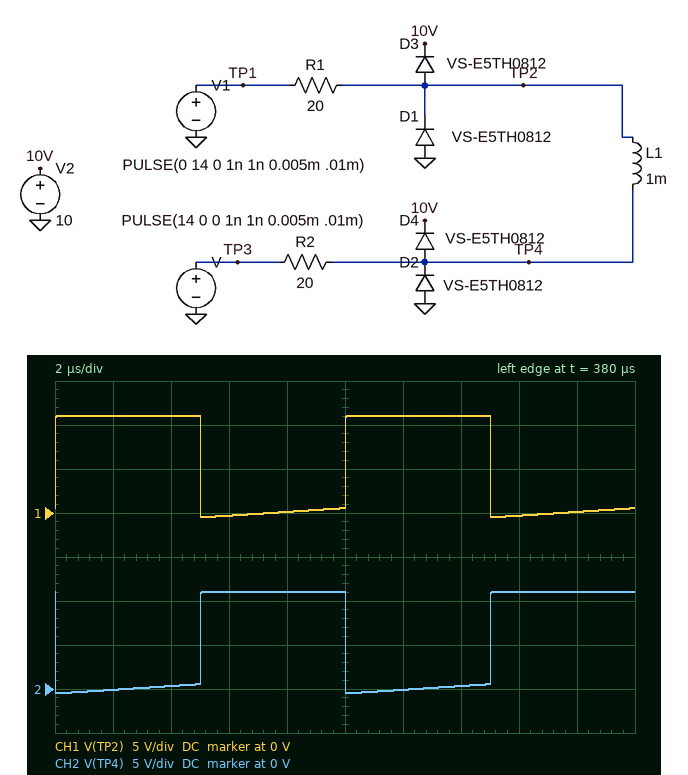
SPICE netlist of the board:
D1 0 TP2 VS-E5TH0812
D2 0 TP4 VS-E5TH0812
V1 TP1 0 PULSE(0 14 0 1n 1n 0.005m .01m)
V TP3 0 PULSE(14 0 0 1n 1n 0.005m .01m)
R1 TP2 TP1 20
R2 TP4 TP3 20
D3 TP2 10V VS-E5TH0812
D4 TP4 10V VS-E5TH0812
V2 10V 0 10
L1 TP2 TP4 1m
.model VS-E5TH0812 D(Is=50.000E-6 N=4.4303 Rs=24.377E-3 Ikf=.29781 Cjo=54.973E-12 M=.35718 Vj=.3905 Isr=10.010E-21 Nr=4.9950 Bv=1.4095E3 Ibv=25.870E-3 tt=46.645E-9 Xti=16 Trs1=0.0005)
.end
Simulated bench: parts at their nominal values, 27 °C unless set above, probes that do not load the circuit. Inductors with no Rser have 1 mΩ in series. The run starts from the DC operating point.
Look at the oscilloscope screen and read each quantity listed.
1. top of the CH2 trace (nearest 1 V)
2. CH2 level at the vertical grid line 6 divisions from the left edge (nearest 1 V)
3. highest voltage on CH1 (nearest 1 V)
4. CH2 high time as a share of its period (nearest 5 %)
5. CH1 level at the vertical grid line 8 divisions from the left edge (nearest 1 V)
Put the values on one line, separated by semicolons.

11 V; 0 V; 11 V; 50 %; 0 V
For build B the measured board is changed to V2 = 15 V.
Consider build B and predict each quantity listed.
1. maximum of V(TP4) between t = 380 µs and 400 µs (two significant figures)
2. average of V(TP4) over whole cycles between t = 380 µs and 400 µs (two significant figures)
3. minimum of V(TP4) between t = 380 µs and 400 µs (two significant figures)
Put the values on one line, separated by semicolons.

15 V; 7.0 V; -560 mV
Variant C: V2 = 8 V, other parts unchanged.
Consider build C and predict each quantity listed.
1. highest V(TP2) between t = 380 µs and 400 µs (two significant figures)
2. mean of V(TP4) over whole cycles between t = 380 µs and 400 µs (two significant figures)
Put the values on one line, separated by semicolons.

9.1 V; 4.6 V
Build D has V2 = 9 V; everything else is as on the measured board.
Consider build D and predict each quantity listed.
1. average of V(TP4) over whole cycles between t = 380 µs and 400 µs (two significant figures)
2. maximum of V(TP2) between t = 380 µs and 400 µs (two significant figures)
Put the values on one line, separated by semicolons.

5.0 V; 10 V
